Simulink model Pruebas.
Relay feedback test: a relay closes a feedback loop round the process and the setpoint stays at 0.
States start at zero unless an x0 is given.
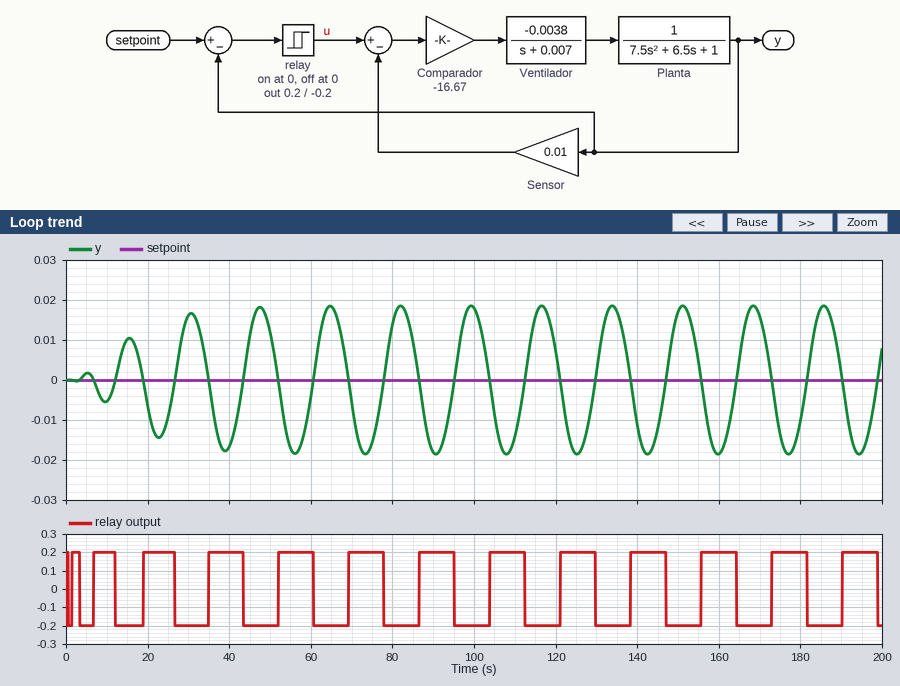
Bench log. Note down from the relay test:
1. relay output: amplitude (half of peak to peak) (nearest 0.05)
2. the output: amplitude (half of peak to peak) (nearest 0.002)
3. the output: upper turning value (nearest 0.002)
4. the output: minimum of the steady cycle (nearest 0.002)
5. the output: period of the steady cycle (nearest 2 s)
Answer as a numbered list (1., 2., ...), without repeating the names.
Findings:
1. 0.20
2. 0.018
3. 0.018
4. -0.018
5. 18 s
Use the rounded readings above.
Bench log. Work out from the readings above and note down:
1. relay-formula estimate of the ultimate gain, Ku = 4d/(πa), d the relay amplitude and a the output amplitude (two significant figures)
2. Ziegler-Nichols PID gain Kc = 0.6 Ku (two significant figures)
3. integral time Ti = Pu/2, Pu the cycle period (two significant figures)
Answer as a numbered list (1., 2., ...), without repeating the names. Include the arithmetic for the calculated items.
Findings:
1. 4 × 0.2 / (π × 0.018) = 14
2. 0.6 × 14 = 8.4
3. 18 / 2 = 9.0 s
